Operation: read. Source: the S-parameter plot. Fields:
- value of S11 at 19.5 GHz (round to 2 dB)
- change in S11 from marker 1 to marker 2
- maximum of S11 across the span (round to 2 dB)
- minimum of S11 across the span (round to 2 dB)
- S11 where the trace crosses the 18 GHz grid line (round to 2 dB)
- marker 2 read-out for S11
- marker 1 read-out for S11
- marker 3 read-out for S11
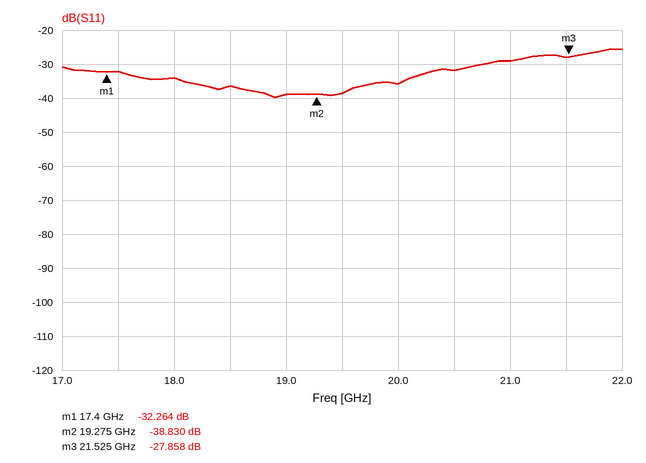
-38 dB
-6.566 dB
-26 dB
-40 dB
-34 dB
-38.830 dB
-32.264 dB
-27.858 dB
